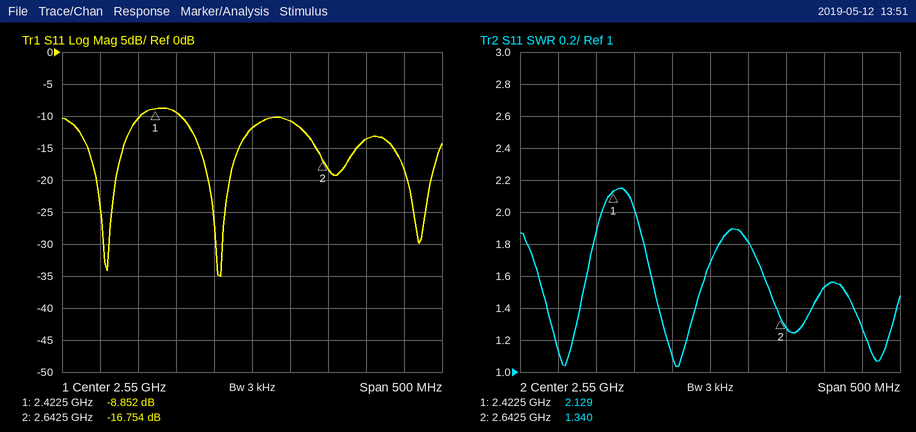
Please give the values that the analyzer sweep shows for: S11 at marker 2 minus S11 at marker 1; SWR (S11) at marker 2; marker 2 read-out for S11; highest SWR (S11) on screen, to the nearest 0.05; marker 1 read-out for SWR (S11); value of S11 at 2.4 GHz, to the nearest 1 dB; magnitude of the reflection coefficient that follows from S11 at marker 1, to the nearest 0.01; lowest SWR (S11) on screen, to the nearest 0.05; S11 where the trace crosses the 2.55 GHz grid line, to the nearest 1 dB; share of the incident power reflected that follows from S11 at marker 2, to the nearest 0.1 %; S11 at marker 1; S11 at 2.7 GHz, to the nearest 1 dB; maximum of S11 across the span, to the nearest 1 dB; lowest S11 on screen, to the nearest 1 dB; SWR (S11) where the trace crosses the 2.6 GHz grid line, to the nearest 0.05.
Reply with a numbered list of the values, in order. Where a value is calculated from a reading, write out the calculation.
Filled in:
1. -16.754 − (-8.852) = -7.902 dB
2. 1.340
3. -16.754 dB
4. 2.15
5. 2.129
6. -10 dB
7. 10^(-8.852/20) ≈ 0.36
8. 1.05
9. -12 dB
10. 10^(-16.754/10) ≈ 2.1 %
11. -8.852 dB
12. -14 dB
13. -9 dB
14. -35 dB
15. 1.80
